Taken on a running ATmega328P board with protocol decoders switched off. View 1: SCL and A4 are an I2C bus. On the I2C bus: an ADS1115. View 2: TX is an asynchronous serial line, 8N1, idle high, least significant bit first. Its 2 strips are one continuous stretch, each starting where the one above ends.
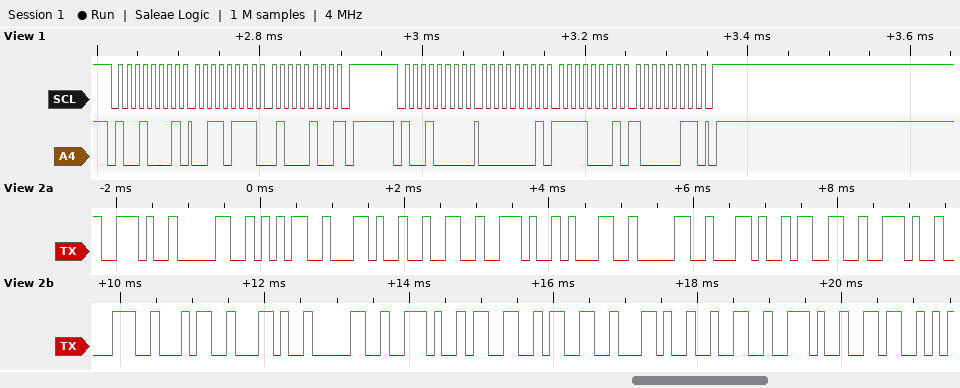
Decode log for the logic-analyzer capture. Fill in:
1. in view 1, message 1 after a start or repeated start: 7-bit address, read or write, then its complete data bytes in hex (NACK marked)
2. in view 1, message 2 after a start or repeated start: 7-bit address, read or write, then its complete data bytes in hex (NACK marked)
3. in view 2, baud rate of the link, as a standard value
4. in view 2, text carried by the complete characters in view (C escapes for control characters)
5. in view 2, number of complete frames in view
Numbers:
0x48 read: 37 44 NACK
0x48 write: 01 F1 83
9600 baud
".05,2.10,3.84,0.33,2.6"
22
